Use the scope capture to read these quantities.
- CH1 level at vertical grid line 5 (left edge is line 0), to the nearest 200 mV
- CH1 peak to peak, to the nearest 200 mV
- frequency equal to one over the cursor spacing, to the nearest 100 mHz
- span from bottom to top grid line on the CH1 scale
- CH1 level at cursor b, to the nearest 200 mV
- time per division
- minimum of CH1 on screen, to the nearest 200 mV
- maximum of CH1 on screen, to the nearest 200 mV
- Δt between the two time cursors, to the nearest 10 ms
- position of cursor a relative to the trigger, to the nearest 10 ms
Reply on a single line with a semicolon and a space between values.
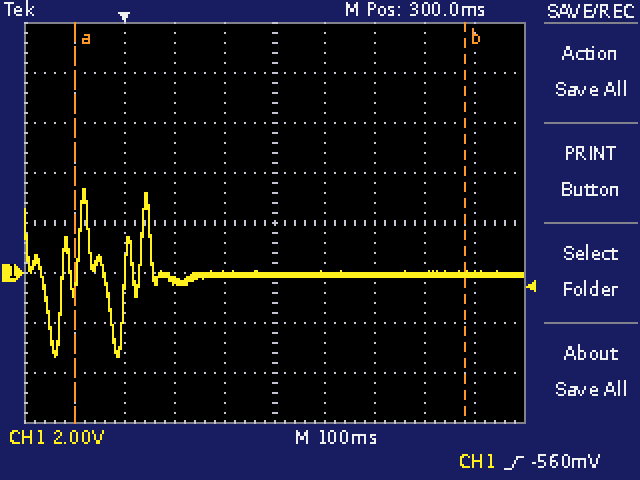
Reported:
0.0 V; 6.8 V; 1.3 Hz; 16 V; 0.0 V; 100 ms; -3.4 V; 3.4 V; 780 ms; -100 ms
